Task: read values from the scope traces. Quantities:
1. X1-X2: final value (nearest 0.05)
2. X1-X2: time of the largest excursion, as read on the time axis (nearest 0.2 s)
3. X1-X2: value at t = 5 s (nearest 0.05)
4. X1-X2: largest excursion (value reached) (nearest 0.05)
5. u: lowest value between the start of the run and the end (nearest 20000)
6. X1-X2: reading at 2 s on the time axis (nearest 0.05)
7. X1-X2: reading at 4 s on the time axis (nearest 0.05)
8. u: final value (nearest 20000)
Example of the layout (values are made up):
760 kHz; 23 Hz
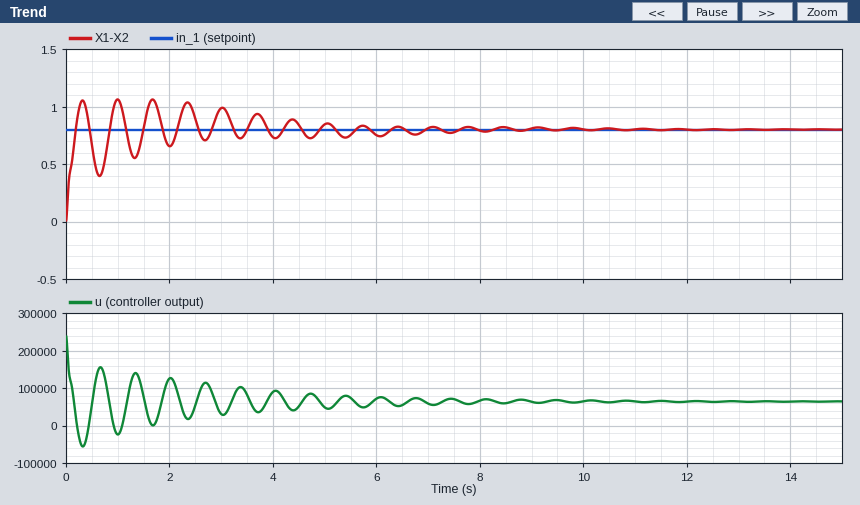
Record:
0.80; 1.0 s; 0.85; 1.05; -60000; 0.65; 0.75; 60000
